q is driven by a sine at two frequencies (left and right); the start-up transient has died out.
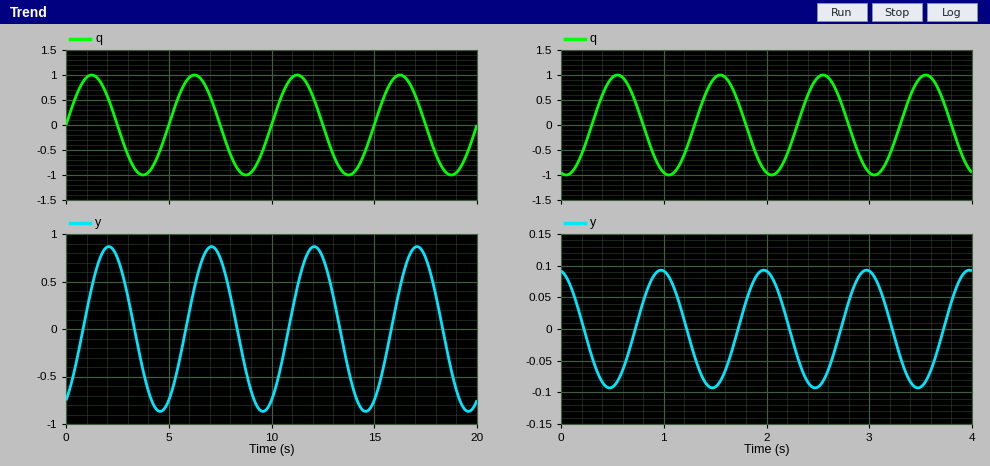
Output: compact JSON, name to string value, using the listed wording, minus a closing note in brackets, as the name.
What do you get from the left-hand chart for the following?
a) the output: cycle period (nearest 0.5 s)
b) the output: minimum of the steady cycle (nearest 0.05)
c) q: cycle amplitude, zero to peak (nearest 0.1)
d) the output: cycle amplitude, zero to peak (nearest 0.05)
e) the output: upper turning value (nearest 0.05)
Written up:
{"the output: cycle period": "5.0 s", "the output: minimum of the steady cycle": "-0.85", "q: cycle amplitude, zero to peak": "1.0", "the output: cycle amplitude, zero to peak": "0.85", "the output: upper turning value": "0.85"}
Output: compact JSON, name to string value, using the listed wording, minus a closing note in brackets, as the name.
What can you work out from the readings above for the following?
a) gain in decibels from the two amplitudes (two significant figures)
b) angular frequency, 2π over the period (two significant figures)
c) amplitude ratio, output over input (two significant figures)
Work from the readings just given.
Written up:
{"gain in decibels from the two amplitudes": "-1.4 dB", "angular frequency, 2π over the period": "1.3 rad/s", "amplitude ratio, output over input": "0.85"}
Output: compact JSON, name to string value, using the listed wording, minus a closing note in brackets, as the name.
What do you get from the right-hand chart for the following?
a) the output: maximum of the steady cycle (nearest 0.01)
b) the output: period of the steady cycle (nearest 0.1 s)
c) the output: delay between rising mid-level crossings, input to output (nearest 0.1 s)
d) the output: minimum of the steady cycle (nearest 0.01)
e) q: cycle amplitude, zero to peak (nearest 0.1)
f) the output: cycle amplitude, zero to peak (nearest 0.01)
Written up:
{"the output: maximum of the steady cycle": "0.09", "the output: period of the steady cycle": "1.0 s", "the output: delay between rising mid-level crossings, input to output": "0.4 s", "the output: minimum of the steady cycle": "-0.09", "q: cycle amplitude, zero to peak": "1.0", "the output: cycle amplitude, zero to peak": "0.09"}
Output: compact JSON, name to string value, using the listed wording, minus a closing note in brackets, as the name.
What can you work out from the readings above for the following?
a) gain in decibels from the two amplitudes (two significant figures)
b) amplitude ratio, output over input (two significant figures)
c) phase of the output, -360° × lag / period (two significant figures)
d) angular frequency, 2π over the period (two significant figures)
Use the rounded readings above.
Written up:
{"gain in decibels from the two amplitudes": "-21 dB", "amplitude ratio, output over input": "0.090", "phase of the output, -360° × lag / period": "-140°", "angular frequency, 2π over the period": "6.3 rad/s"}
